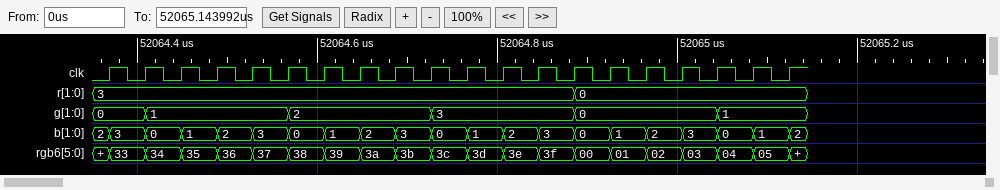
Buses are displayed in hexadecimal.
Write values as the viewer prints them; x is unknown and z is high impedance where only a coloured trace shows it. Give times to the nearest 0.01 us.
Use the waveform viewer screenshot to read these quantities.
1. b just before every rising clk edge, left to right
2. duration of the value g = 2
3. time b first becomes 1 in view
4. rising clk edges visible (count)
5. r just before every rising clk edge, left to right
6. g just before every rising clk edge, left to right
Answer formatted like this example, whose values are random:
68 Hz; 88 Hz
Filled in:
2, 3, 0, 1, 2, 3, 0, 1, 2, 3, 0, 1, 2, 3, 0, 1, 2, 3, 0, 1; 0.16 us; 52064.45 us; 20; 3, 3, 3, 3, 3, 3, 3, 3, 3, 3, 3, 3, 3, 3, 0, 0, 0, 0, 0, 0; 0, 0, 1, 1, 1, 1, 2, 2, 2, 2, 3, 3, 3, 3, 0, 0, 0, 0, 1, 1
